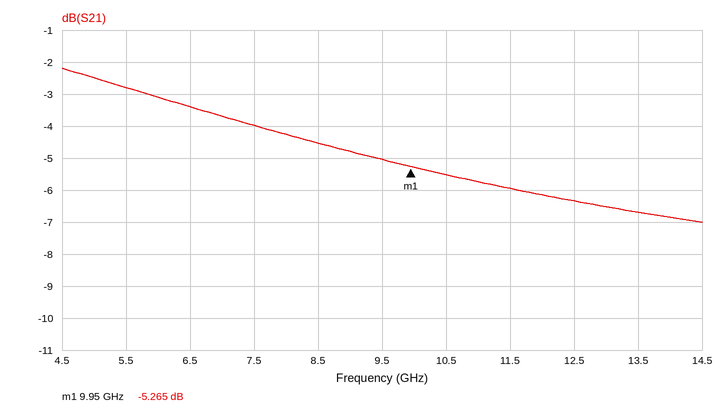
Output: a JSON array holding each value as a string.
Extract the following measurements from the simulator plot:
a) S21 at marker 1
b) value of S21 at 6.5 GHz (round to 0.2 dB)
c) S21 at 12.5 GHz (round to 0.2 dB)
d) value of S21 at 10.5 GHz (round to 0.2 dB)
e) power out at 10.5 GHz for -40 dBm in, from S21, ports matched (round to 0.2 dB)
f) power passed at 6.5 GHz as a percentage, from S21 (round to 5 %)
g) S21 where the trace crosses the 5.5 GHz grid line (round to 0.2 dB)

["-5.265 dB", "-3.4 dB", "-6.4 dB", "-5.6 dB", "-45.6 dBm", "45 %", "-2.8 dB"]
